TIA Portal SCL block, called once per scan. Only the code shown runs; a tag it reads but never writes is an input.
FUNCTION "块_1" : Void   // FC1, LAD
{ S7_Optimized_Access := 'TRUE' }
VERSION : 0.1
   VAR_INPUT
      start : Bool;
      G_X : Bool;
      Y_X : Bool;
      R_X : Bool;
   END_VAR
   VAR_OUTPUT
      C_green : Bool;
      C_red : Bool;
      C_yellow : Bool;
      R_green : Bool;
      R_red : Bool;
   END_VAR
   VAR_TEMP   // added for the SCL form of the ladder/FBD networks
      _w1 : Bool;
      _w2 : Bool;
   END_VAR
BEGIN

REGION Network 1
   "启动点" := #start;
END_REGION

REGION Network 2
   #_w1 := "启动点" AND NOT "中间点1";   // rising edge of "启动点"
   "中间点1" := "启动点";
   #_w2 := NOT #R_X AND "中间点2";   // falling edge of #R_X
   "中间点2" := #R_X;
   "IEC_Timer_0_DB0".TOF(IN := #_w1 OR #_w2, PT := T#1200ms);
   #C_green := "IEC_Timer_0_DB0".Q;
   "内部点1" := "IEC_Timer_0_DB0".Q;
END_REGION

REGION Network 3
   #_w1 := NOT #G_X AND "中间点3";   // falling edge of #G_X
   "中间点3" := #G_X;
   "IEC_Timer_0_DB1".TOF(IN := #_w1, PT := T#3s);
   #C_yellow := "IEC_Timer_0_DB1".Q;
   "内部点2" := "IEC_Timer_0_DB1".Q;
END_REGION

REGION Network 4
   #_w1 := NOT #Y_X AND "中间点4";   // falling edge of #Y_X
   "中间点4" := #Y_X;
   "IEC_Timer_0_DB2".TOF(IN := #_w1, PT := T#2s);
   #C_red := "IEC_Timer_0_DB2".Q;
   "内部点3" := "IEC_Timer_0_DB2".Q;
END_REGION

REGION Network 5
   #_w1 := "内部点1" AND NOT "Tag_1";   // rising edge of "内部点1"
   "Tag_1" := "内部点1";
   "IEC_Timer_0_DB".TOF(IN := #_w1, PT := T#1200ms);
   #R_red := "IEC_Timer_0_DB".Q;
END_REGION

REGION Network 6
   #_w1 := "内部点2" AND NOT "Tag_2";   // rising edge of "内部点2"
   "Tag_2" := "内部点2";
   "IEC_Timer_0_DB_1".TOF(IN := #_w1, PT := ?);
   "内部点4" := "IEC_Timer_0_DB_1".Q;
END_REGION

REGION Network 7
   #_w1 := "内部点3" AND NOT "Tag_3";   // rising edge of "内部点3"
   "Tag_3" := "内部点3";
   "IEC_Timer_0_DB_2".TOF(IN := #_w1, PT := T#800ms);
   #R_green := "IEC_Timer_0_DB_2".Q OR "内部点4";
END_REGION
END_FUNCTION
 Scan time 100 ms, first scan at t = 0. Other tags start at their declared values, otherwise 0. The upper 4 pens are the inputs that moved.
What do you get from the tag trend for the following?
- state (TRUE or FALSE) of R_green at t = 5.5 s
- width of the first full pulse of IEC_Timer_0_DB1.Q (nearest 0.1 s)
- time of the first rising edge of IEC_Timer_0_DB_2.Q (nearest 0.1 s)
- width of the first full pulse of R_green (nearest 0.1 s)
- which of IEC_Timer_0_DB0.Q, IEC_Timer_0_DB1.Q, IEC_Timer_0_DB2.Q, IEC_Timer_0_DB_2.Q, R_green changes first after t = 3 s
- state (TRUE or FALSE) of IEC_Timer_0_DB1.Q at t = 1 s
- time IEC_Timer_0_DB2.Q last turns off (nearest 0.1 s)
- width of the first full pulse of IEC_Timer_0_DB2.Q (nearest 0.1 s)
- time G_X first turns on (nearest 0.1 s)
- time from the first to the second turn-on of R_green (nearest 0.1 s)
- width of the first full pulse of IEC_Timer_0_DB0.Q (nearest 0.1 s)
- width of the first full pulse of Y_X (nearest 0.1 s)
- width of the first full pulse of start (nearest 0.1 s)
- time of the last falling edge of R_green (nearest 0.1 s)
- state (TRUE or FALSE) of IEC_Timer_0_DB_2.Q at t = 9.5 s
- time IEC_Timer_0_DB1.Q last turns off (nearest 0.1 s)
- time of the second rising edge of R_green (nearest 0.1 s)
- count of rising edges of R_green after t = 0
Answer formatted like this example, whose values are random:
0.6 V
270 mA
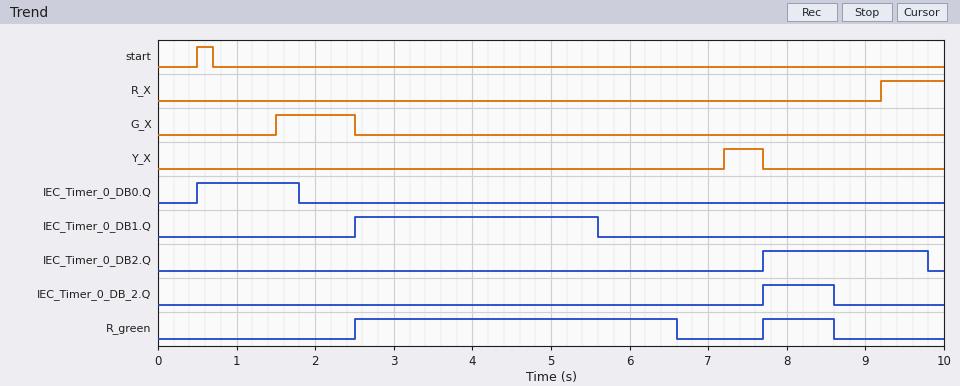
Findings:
TRUE
3.1 s
7.7 s
4.1 s
IEC_Timer_0_DB1.Q
FALSE
9.8 s
2.1 s
1.5 s
5.2 s
1.3 s
0.5 s
0.2 s
8.6 s
FALSE
5.6 s
7.7 s
2
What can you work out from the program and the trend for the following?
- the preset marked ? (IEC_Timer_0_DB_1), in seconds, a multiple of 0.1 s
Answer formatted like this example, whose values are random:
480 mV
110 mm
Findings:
4.0 s
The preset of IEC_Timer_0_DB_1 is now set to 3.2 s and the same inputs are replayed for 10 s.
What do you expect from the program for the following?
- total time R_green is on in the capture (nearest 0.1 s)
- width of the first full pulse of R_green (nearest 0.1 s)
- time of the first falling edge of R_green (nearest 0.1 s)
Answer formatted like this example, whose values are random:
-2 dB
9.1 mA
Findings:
4.2 s
3.3 s
5.8 s
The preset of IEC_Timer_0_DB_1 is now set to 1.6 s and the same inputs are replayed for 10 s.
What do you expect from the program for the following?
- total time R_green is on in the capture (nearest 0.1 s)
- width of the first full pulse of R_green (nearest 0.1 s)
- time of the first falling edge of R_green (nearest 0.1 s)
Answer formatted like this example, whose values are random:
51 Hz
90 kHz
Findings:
2.6 s
1.7 s
4.2 s
